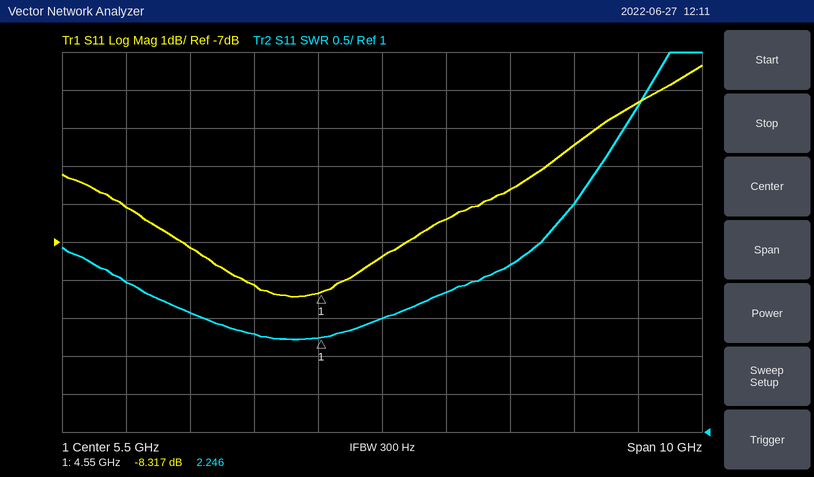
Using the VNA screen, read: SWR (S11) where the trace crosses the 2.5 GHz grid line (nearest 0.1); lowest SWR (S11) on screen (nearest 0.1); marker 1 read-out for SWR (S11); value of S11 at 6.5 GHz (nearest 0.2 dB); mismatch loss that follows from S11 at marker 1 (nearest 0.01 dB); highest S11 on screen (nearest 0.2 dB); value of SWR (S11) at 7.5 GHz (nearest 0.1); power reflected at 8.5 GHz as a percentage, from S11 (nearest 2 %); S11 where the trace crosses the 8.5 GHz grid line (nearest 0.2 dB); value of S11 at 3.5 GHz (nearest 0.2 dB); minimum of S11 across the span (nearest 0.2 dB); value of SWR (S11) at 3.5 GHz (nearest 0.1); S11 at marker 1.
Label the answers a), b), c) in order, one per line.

a) 2.6
b) 2.2
c) 2.246
d) -6.4 dB
e) 0.69 dB
f) -2.4 dB
g) 3.2
h) 36 %
i) -4.4 dB
j) -8.2 dB
k) -8.4 dB
l) 2.3
m) -8.317 dB
